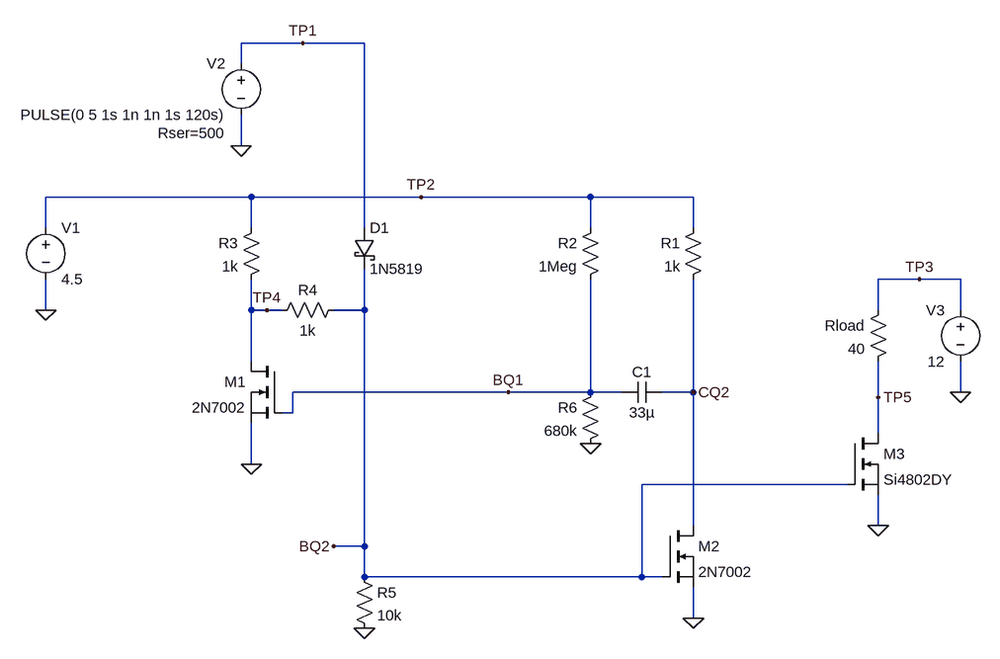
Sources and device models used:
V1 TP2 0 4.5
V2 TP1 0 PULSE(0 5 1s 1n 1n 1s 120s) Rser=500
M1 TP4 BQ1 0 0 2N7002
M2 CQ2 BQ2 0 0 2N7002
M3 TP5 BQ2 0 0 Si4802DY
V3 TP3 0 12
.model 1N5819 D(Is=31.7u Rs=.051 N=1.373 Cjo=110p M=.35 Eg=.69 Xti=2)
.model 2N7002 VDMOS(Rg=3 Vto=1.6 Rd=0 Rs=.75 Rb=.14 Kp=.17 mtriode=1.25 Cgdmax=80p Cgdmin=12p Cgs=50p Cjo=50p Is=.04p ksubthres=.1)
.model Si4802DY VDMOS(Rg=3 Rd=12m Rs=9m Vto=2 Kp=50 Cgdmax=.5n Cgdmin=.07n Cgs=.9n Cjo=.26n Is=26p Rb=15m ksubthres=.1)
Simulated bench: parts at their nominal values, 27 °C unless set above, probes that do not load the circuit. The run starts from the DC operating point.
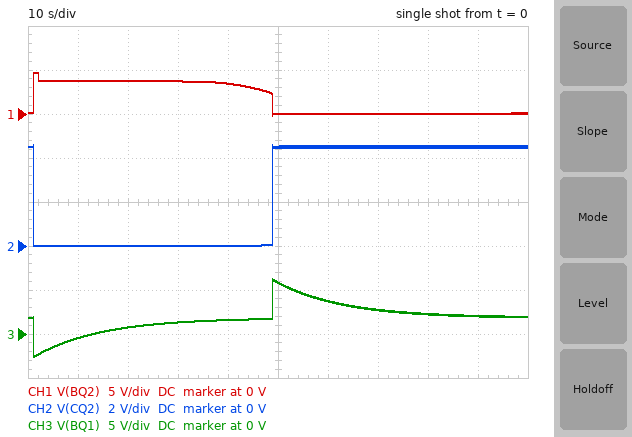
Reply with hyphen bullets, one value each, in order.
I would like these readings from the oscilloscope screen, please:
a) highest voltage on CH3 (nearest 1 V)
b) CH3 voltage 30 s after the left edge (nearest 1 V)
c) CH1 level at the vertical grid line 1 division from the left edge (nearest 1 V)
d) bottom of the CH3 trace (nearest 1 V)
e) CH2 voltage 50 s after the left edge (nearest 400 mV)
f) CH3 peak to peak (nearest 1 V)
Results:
- 6 V
- 1 V
- 4 V
- -3 V
- 4.4 V
- 9 V
